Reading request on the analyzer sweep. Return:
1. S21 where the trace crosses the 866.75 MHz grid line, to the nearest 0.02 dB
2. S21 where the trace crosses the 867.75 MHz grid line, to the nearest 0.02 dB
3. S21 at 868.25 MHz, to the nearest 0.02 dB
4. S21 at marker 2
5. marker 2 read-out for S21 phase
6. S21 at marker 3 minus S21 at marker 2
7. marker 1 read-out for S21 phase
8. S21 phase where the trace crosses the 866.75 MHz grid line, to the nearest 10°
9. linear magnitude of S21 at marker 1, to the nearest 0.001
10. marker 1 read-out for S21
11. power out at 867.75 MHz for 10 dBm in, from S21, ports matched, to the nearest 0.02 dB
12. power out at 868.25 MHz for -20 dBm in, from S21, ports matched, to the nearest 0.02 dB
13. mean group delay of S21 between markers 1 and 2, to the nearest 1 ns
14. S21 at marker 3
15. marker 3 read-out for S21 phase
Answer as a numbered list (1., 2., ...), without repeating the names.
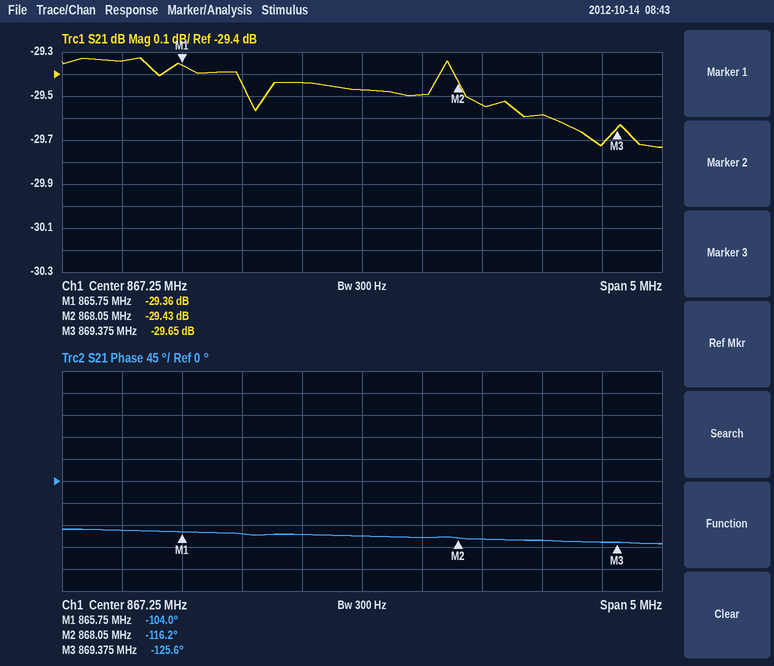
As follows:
1. -29.44 dB
2. -29.50 dB
3. -29.54 dB
4. -29.43 dB
5. -116.2°
6. -0.22 dB
7. -104.0°
8. -110°
9. 0.034
10. -29.36 dB
11. -19.50 dBm
12. -49.54 dBm
13. 15 ns
14. -29.65 dB
15. -125.6°
